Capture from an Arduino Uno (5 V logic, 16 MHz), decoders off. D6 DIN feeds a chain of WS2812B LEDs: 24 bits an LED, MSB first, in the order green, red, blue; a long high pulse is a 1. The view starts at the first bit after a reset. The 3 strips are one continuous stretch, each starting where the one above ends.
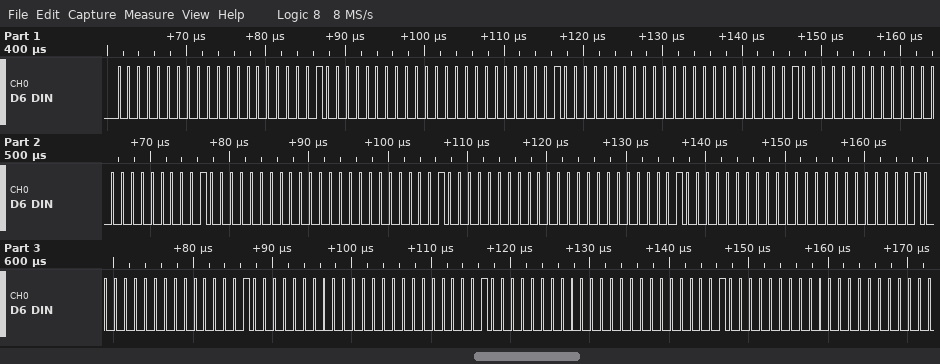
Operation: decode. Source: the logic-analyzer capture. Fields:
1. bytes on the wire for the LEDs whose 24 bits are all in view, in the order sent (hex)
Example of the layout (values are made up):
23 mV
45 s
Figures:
00 00 08 00 00 08 00 00 08 00 00 08 00 00 08 00 00 08 00 00 08 00 08 00 00 08 00 00 08 00
